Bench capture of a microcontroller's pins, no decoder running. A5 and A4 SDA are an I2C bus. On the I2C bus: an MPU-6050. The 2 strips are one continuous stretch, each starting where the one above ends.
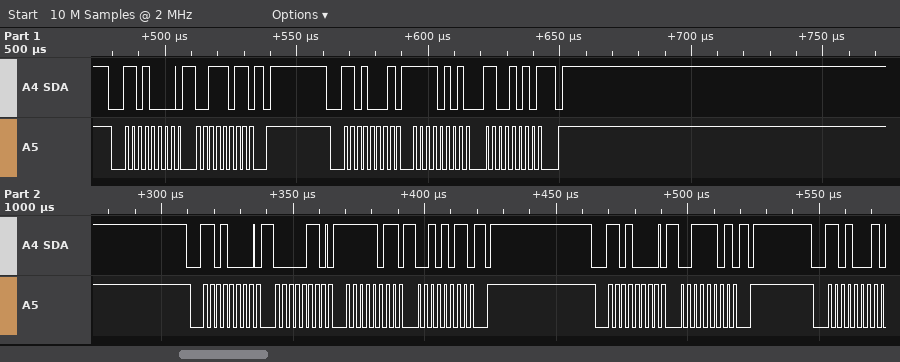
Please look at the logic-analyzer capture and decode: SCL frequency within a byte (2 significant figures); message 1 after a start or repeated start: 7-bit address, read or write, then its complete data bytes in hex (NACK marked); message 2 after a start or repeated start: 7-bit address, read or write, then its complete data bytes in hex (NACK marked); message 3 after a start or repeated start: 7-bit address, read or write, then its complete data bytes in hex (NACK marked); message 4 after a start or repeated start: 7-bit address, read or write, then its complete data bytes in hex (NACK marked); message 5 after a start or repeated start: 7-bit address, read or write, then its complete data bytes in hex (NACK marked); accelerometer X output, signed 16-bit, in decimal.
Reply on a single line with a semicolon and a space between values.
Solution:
400 kHz; 0x68 write: 3B; 0x68 read: F5 CA NACK; 0x68 write: 06 FB 2B; 0x68 write: 3D; 0x68 read; -2614
